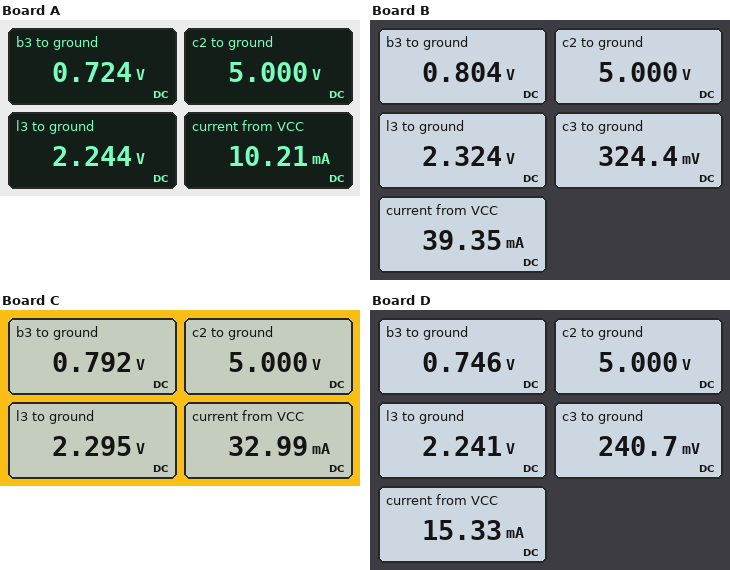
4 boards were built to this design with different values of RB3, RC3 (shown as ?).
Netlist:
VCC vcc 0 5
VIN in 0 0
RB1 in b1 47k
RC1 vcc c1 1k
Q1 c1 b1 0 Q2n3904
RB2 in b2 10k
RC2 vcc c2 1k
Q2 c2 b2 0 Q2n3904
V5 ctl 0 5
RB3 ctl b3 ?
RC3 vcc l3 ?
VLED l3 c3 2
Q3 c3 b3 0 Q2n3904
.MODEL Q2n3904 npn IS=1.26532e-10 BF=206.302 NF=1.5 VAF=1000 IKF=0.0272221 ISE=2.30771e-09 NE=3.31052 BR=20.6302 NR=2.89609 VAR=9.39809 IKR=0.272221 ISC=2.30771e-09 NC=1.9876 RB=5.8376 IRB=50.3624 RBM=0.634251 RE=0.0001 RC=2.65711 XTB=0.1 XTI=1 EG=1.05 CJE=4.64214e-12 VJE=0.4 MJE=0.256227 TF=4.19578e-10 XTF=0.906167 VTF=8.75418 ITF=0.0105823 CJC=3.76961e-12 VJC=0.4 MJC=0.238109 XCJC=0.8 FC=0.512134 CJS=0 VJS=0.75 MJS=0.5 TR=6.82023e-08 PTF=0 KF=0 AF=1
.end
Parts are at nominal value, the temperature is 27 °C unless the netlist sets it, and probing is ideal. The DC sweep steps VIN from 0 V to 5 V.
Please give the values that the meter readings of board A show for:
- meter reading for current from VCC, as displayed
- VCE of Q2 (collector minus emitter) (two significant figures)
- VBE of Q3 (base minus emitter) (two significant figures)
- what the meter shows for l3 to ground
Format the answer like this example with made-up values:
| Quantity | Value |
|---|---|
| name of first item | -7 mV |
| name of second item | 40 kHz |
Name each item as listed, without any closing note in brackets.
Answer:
| Quantity | Value |
|---|---|
| meter reading for current from VCC, as displayed | 10.21 mA |
| VCE of Q2 (collector minus emitter) | 5.0 V |
| VBE of Q3 (base minus emitter) | 720 mV |
| what the meter shows for l3 to ground | 2.244 V |
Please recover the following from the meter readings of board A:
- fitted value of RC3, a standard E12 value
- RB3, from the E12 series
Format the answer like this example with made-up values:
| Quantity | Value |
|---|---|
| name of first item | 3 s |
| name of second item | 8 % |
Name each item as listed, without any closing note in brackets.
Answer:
| Quantity | Value |
|---|---|
| fitted value of RC3, a standard E12 value | 270 Ω |
| RB3, from the E12 series | 33 kΩ |
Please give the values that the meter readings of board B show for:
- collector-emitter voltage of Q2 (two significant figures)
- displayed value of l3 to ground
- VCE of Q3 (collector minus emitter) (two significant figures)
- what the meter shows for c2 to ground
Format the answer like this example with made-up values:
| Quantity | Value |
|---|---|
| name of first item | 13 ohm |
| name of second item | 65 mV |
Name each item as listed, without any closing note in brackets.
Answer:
| Quantity | Value |
|---|---|
| collector-emitter voltage of Q2 | 5.0 V |
| displayed value of l3 to ground | 2.324 V |
| VCE of Q3 (collector minus emitter) | 320 mV |
| what the meter shows for c2 to ground | 5.000 V |
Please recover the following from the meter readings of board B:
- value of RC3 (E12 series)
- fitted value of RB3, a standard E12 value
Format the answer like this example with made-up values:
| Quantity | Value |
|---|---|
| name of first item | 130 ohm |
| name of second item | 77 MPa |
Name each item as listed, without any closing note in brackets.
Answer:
| Quantity | Value |
|---|---|
| value of RC3 | 68 Ω |
| fitted value of RB3, a standard E12 value | 5.6 kΩ |
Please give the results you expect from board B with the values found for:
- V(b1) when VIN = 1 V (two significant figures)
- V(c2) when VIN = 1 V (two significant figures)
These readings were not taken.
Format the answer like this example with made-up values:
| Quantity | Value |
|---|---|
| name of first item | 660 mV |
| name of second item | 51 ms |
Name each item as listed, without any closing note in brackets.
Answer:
| Quantity | Value |
|---|---|
| V(b1) when VIN = 1 V | 620 mV |
| V(c2) when VIN = 1 V | 830 mV |
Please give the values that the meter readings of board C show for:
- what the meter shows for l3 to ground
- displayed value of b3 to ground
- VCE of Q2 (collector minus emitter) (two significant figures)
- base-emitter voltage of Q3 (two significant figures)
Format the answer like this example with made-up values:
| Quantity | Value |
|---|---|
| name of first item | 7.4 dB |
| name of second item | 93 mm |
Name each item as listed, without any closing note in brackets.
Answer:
| Quantity | Value |
|---|---|
| what the meter shows for l3 to ground | 2.295 V |
| displayed value of b3 to ground | 0.792 V |
| VCE of Q2 (collector minus emitter) | 5.0 V |
| base-emitter voltage of Q3 | 790 mV |
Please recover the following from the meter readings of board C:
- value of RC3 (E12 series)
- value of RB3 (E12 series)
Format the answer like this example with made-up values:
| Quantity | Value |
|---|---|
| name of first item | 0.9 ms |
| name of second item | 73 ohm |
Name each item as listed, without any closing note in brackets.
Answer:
| Quantity | Value |
|---|---|
| value of RC3 | 82 Ω |
| value of RB3 | 6.8 kΩ |
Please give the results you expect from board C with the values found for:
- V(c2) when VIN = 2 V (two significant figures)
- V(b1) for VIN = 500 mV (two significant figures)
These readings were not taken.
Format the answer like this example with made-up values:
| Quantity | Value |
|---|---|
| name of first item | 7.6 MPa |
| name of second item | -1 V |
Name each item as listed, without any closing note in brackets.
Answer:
| Quantity | Value |
|---|---|
| V(c2) when VIN = 2 V | 160 mV |
| V(b1) for VIN = 500 mV | 470 mV |
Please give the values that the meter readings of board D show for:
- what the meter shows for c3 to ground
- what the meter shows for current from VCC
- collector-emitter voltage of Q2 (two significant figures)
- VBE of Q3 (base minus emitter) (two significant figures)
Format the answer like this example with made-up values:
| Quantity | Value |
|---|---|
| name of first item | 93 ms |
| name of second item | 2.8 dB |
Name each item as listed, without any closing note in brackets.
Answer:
| Quantity | Value |
|---|---|
| what the meter shows for c3 to ground | 240.7 mV |
| what the meter shows for current from VCC | 15.33 mA |
| collector-emitter voltage of Q2 | 5.0 V |
| VBE of Q3 (base minus emitter) | 750 mV |
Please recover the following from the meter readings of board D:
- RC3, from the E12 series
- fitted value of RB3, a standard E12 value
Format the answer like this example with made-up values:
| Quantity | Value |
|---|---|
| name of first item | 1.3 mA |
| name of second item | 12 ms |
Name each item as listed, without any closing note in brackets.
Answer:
| Quantity | Value |
|---|---|
| RC3, from the E12 series | 180 Ω |
| fitted value of RB3, a standard E12 value | 18 kΩ |
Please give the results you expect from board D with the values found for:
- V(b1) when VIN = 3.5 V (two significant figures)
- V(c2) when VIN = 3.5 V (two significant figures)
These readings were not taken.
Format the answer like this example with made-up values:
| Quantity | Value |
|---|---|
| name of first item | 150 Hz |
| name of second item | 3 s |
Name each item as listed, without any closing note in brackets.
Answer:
| Quantity | Value |
|---|---|
| V(b1) when VIN = 3.5 V | 690 mV |
| V(c2) when VIN = 3.5 V | 110 mV |
